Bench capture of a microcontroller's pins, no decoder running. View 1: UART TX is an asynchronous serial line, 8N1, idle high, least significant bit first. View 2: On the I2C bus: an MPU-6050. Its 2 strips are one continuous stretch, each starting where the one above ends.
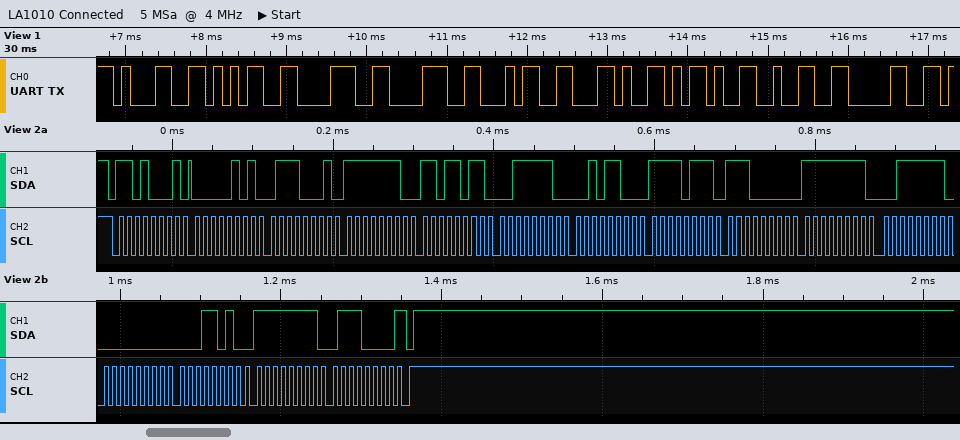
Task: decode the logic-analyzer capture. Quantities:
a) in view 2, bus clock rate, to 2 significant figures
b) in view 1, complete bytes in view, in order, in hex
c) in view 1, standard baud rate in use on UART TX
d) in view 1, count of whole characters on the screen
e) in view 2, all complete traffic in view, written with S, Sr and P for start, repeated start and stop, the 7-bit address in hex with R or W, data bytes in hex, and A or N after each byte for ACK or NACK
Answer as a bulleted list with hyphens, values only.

- 100 kHz
- 31 35 38 38 34 2C 2D 32 30
- 9600 baud
- 9
- S 68R A 05 A 71 A FE A DB A 3E A 2C A F7 A E0 A FF A 3F A 00 A 1A A FF A 70 N P
